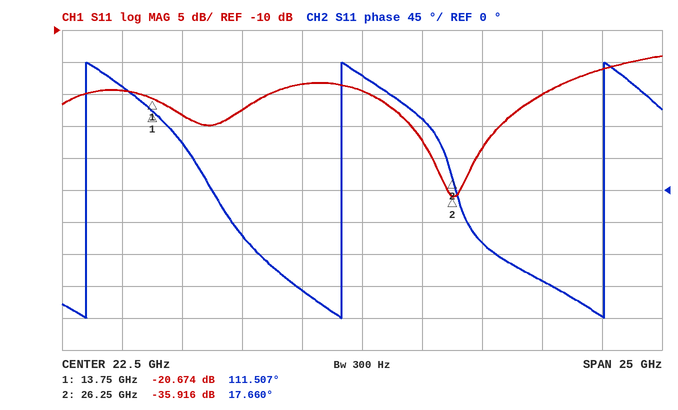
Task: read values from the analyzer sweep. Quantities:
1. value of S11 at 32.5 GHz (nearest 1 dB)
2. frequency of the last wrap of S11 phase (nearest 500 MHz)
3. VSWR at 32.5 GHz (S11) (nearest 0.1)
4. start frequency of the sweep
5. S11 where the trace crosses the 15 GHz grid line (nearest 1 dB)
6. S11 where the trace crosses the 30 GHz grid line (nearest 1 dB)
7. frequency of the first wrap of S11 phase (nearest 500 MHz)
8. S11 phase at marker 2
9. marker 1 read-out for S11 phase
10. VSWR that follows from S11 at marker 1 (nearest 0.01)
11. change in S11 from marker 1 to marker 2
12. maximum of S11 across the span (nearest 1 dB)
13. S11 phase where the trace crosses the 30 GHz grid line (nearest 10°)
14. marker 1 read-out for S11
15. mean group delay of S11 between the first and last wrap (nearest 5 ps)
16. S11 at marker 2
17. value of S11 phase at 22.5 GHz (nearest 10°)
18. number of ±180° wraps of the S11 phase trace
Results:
-16 dB
32.5 GHz
1.4
10 GHz
-23 dB
-20 dB
11.0 GHz
17.660°
111.507°
1.20
-15.242 dB
-14 dB
-130°
-20.674 dB
95 ps
-35.916 dB
160°
3
